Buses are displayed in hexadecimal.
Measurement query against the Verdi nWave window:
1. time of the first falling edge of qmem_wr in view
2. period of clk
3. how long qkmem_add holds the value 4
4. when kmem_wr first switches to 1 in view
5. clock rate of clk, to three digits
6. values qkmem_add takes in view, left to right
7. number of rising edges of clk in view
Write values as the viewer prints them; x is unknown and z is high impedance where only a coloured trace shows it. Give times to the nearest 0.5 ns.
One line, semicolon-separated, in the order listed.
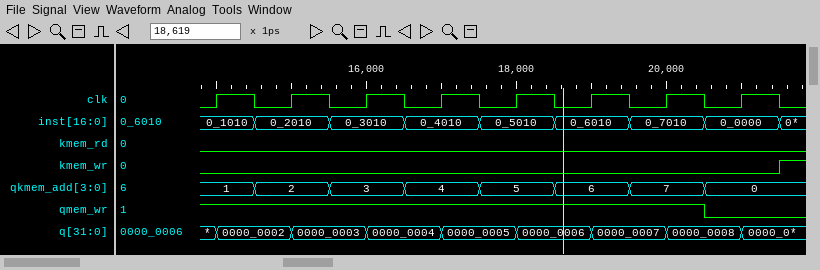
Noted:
20.5 ns; 1 ns; 1 ns; 21.5 ns; 1.00 GHz; 1, 2, 3, 4, 5, 6, 7, 0; 8
